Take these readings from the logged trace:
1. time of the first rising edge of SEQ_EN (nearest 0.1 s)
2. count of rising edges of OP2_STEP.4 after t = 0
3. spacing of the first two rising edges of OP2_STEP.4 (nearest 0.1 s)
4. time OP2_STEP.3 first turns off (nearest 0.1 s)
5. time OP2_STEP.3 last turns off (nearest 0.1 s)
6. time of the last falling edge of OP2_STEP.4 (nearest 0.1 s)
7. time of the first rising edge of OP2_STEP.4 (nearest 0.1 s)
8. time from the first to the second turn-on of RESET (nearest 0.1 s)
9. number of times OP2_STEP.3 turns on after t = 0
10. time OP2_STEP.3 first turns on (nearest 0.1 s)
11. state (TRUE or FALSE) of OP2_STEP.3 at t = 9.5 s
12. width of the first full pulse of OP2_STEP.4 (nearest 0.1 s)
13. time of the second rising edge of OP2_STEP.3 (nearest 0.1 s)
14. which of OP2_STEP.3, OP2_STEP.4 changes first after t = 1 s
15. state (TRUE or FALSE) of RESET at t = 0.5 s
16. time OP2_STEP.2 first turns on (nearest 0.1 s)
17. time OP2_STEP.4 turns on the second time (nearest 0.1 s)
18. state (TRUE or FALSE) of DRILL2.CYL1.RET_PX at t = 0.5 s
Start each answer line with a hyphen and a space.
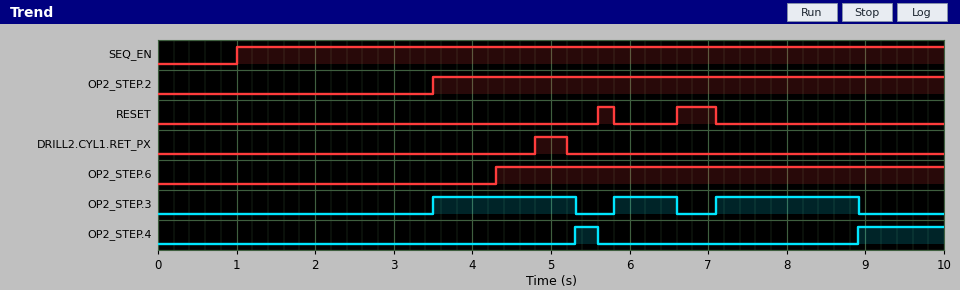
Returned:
- 1.0 s
- 2
- 3.6 s
- 5.3 s
- 8.9 s
- 5.6 s
- 5.3 s
- 1.0 s
- 3
- 3.5 s
- FALSE
- 0.3 s
- 5.8 s
- OP2_STEP.3
- FALSE
- 3.5 s
- 8.9 s
- FALSE
